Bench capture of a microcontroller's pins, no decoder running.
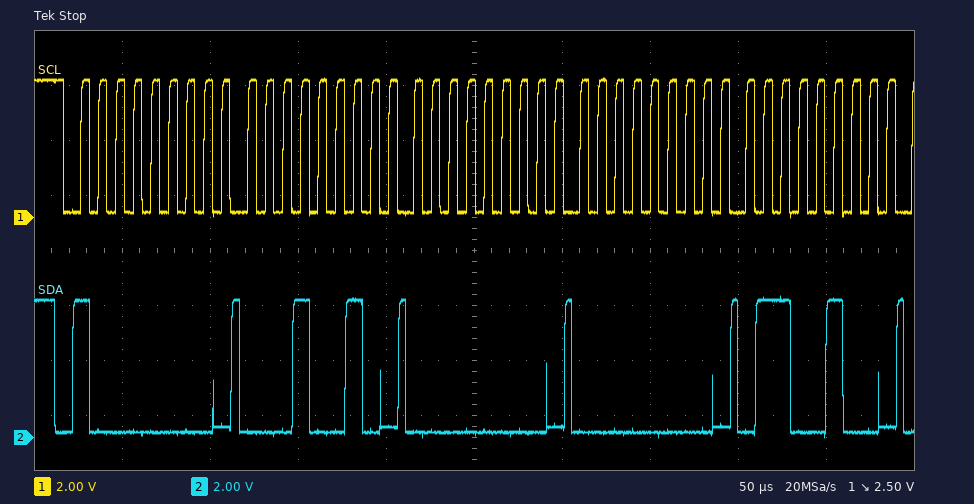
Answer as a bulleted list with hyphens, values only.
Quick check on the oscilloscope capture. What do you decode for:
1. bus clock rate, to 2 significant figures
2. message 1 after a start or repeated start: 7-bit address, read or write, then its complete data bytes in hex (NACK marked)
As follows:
- 100 kHz
- 0x40 write: 12 00 00 64
